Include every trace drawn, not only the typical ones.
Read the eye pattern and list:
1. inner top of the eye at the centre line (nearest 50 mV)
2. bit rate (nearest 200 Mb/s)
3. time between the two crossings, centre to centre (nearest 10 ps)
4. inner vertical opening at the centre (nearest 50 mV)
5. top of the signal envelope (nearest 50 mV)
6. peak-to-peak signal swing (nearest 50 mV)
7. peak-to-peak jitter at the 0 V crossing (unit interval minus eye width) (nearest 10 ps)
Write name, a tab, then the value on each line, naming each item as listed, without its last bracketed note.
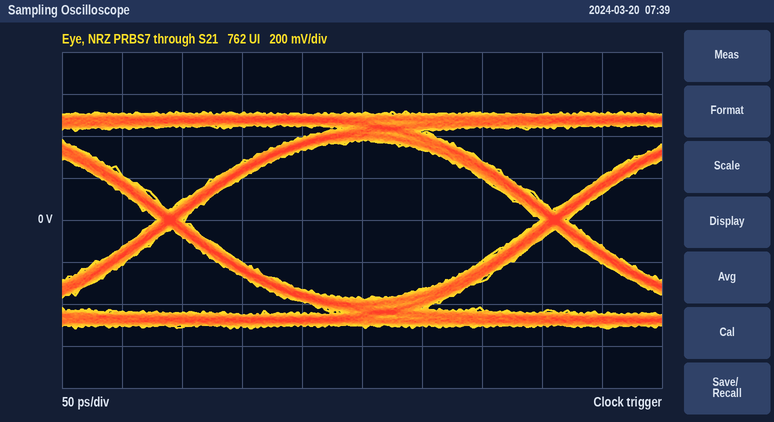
inner top of the eye at the centre line	400 mV
bit rate	3.2 Gb/s
time between the two crossings, centre to centre	320 ps
inner vertical opening at the centre	750 mV
top of the signal envelope	500 mV
peak-to-peak signal swing	1.05 V
peak-to-peak jitter at the 0 V crossing (unit interval minus eye width)	20 ps
